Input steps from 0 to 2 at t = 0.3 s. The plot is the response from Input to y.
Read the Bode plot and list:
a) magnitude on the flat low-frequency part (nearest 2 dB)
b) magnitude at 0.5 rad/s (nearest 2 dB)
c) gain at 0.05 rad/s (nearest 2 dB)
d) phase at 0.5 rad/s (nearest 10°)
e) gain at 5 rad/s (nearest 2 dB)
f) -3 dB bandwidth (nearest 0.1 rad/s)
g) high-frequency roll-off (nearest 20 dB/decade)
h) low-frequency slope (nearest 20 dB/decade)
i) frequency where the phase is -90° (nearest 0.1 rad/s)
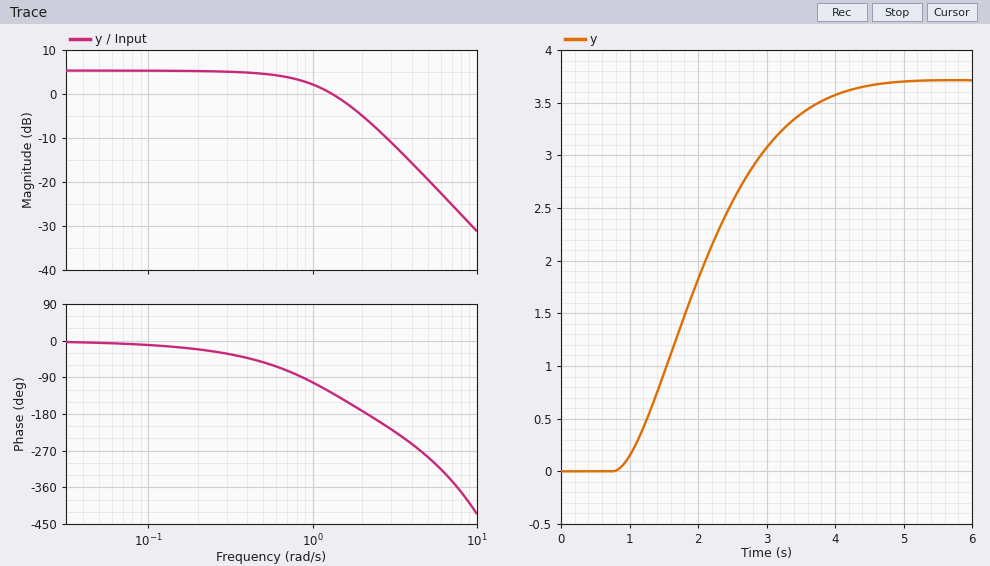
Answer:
6 dB
4 dB
6 dB
-50°
-20 dB
1.0 rad/s
-40 dB/decade
0 dB/decade
0.9 rad/s
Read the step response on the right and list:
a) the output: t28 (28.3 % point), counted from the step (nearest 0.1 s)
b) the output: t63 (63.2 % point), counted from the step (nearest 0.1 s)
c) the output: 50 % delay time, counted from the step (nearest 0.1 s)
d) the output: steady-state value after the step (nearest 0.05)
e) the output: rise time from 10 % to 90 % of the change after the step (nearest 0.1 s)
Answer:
1.3 s
2.0 s
1.7 s
3.70
2.2 s
